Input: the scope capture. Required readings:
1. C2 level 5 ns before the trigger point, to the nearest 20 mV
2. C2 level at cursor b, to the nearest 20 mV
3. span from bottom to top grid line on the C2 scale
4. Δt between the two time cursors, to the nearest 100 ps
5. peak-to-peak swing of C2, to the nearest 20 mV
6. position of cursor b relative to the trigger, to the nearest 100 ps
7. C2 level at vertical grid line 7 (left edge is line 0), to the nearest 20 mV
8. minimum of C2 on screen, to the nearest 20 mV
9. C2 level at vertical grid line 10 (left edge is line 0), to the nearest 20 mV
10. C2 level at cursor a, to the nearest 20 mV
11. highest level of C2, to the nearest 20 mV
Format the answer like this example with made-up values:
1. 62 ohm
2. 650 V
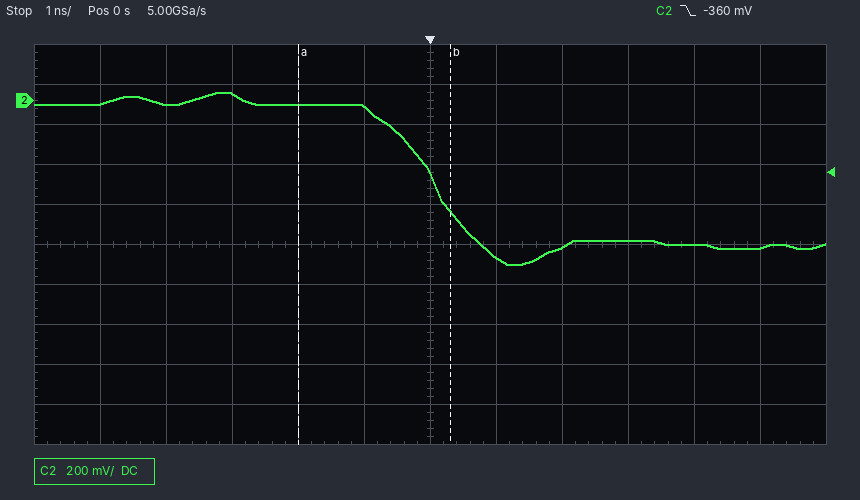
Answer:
1. -20 mV
2. -560 mV
3. 2 V
4. 2.3 ns
5. 860 mV
6. +300 ps
7. -780 mV
8. -820 mV
9. -720 mV
10. -20 mV
11. 40 mV
